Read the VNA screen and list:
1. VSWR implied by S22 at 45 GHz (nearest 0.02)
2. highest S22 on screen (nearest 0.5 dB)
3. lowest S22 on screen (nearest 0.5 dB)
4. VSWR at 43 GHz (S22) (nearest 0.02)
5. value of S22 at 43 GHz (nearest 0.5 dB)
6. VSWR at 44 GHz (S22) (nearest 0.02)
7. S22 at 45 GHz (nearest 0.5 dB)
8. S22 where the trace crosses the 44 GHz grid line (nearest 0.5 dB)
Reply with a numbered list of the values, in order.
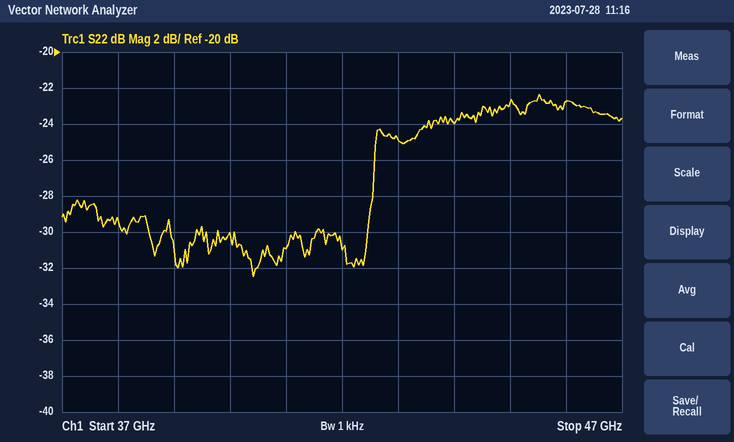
1. 1.16
2. -22.5 dB
3. -32.5 dB
4. 1.12
5. -25.0 dB
6. 1.14
7. -23.0 dB
8. -24.0 dB
